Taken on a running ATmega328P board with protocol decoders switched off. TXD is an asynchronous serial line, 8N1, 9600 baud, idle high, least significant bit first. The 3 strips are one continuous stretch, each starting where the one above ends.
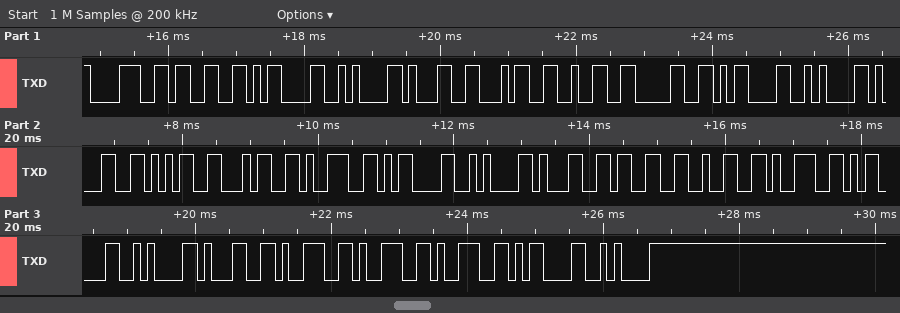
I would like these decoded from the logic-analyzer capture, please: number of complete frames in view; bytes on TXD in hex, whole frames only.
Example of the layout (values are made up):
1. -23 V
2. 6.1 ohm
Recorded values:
1. 28
2. 38 33 0D 0A 31 34 32 30 0D 0A 31 35 34 39 0D 0A 31 33 32 39 0D 0A 31 39 39 39 0D 0A
